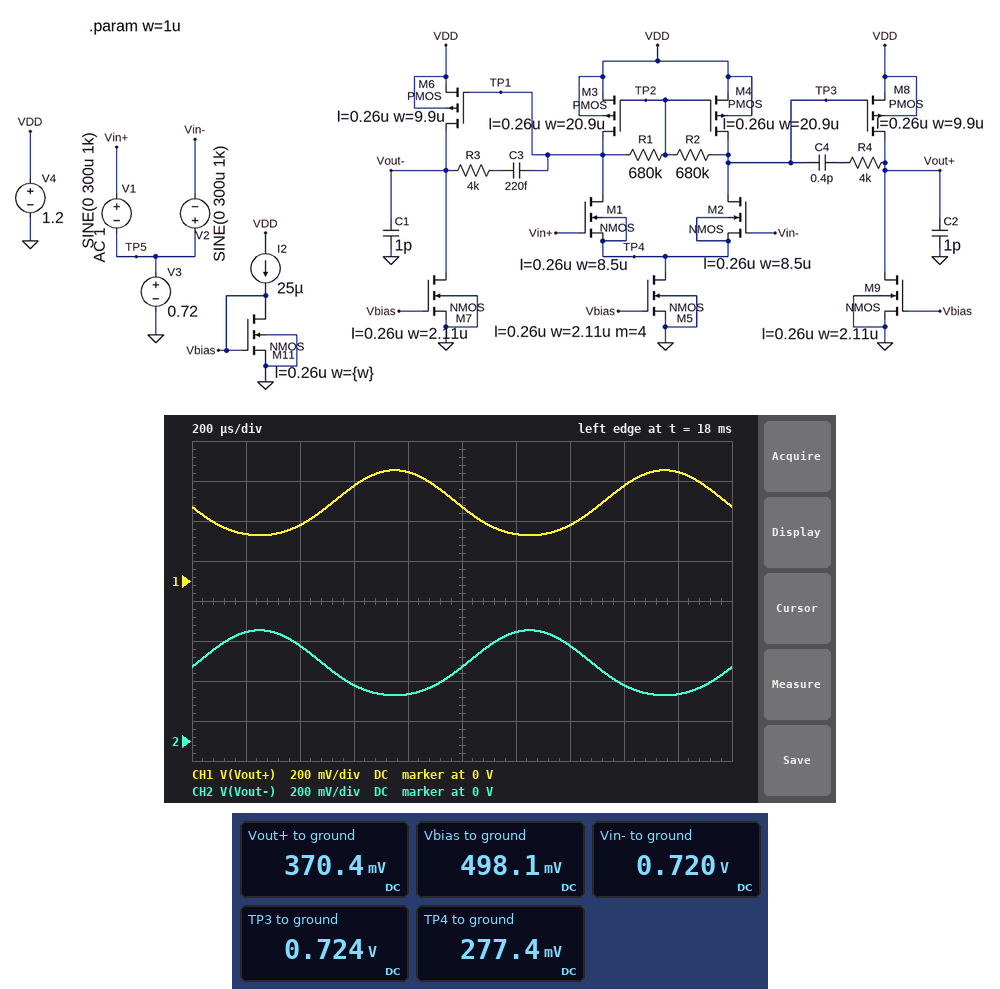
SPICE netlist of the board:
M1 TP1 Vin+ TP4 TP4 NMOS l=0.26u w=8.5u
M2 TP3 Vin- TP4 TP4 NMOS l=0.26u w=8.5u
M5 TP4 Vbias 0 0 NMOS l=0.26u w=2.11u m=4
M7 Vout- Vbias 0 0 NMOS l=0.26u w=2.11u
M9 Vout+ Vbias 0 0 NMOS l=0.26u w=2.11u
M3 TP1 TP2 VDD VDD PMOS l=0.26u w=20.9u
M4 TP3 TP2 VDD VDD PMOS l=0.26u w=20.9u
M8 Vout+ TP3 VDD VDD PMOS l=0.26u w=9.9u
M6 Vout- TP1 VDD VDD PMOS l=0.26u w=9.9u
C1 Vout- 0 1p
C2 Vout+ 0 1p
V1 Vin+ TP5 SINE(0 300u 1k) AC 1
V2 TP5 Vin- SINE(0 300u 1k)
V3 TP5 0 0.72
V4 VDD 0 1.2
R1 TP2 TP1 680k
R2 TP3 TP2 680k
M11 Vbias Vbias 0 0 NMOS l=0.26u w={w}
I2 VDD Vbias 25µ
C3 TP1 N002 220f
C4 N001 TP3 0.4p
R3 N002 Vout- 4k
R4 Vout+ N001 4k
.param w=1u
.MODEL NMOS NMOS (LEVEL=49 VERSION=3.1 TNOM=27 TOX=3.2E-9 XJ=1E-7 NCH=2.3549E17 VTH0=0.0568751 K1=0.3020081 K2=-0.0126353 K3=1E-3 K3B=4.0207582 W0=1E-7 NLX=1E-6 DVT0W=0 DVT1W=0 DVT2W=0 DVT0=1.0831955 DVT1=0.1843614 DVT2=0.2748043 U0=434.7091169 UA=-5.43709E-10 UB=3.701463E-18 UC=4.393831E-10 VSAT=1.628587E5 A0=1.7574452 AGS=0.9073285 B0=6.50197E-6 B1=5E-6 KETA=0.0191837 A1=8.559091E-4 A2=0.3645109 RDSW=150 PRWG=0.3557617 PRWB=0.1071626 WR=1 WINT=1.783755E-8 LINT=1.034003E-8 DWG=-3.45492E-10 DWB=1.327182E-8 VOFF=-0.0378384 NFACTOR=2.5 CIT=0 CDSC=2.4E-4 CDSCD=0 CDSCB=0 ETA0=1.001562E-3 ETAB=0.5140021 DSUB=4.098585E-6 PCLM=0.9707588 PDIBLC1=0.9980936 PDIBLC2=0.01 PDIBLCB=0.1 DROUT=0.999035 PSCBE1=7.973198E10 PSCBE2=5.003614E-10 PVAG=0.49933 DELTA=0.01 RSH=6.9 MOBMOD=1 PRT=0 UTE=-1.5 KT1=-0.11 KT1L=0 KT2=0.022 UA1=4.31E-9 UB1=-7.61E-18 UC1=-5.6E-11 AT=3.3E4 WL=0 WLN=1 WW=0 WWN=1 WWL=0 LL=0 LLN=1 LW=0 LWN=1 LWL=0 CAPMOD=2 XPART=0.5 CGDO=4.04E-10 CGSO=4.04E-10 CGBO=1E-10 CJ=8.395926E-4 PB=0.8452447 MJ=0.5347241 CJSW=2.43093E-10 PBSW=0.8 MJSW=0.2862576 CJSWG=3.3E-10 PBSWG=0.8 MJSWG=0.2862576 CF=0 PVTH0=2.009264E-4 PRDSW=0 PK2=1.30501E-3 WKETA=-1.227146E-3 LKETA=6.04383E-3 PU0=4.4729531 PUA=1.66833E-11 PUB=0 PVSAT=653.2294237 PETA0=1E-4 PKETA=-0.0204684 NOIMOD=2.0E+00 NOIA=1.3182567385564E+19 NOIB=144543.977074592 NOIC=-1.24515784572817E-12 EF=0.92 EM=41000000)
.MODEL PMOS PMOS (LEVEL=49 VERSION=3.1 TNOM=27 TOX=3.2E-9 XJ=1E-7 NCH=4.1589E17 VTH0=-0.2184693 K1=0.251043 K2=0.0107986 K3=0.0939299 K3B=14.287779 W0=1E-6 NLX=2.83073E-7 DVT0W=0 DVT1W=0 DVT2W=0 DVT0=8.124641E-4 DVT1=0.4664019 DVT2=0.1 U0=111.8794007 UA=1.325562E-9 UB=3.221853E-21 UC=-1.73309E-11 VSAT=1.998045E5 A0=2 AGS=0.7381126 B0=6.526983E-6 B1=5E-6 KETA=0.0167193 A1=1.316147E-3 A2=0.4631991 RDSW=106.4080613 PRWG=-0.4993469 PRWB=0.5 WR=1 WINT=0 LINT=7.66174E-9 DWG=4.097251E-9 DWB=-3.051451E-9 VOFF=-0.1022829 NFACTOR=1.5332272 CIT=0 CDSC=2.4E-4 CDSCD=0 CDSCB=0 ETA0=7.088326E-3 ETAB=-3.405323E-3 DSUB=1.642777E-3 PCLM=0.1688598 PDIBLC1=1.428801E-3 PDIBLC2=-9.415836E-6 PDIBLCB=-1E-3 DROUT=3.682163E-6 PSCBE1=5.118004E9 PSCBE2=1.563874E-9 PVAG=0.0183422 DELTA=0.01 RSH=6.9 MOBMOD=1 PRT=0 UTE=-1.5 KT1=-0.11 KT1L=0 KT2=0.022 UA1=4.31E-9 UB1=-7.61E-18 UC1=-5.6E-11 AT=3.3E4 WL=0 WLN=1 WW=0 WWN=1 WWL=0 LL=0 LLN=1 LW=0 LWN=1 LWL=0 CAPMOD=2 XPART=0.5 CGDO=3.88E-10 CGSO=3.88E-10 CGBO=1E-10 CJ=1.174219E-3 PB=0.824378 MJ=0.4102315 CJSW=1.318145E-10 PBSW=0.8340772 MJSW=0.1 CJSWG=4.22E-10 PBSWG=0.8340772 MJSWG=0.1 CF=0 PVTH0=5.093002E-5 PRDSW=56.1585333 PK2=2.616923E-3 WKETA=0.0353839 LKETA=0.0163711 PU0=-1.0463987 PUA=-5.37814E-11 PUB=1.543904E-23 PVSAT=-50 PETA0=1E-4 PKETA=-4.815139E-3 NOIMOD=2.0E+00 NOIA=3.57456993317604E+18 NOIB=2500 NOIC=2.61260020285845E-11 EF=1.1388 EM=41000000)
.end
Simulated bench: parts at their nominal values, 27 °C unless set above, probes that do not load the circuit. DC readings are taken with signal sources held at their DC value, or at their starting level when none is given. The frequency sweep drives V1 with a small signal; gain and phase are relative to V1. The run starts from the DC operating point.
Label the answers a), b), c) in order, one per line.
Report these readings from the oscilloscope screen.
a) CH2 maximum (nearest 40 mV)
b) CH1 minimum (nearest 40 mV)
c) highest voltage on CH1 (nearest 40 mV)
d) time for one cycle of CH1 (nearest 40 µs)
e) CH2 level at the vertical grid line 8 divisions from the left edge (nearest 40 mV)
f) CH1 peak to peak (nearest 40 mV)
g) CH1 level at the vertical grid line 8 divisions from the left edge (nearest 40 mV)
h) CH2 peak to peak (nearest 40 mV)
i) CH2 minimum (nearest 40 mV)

a) 560 mV
b) 240 mV
c) 560 mV
d) 1.00 ms
e) 280 mV
f) 320 mV
g) 480 mV
h) 320 mV
i) 240 mV
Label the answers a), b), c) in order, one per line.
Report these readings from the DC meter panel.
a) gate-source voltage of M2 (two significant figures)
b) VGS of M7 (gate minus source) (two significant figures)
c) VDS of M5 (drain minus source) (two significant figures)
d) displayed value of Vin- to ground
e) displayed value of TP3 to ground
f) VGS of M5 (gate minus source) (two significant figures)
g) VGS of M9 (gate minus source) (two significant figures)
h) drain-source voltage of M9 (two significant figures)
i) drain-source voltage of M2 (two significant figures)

a) 440 mV
b) 500 mV
c) 280 mV
d) 0.720 V
e) 0.724 V
f) 500 mV
g) 500 mV
h) 370 mV
i) 450 mV
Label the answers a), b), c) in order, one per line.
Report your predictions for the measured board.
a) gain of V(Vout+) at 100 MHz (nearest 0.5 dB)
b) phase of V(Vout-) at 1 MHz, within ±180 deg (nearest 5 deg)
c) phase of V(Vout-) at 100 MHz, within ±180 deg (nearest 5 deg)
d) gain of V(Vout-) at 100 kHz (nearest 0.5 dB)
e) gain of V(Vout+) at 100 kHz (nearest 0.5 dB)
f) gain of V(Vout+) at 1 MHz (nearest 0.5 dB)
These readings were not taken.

a) 5.5 dB
b) -45 deg
c) -120 deg
d) 49.0 dB
e) 49.0 dB
f) 46.0 dB
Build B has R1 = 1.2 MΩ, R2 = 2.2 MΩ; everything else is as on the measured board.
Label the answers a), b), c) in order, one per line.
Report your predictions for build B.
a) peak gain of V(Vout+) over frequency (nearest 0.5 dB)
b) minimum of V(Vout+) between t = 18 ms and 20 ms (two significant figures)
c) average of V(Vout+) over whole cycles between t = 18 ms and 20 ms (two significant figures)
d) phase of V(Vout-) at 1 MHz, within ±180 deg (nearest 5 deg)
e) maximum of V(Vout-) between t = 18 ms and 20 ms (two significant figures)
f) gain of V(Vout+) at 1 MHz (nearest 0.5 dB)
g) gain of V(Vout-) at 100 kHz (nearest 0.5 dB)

a) 51.5 dB
b) 200 mV
c) 390 mV
d) -40 deg
e) 500 mV
f) 48.0 dB
g) 46.0 dB
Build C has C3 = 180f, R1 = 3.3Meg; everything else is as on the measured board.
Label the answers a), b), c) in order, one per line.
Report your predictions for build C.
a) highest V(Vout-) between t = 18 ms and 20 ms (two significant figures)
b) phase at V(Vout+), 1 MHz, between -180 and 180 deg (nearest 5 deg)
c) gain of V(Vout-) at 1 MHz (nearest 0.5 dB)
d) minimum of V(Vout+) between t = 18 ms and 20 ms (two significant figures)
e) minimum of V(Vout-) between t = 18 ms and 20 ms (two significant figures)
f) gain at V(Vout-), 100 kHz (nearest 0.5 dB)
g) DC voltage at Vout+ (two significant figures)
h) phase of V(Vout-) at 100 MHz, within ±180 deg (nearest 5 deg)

a) 680 mV
b) 145 deg
c) 51.5 dB
d) 310 mV
e) 170 mV
f) 53.5 dB
g) 370 mV
h) -125 deg
